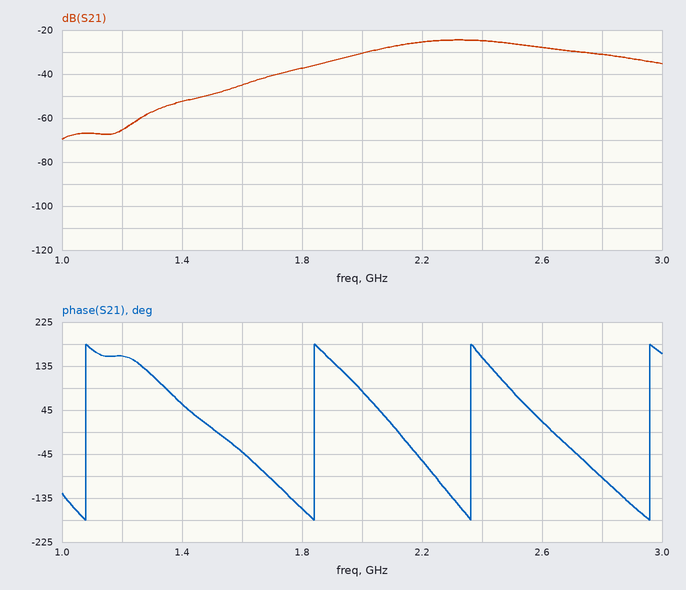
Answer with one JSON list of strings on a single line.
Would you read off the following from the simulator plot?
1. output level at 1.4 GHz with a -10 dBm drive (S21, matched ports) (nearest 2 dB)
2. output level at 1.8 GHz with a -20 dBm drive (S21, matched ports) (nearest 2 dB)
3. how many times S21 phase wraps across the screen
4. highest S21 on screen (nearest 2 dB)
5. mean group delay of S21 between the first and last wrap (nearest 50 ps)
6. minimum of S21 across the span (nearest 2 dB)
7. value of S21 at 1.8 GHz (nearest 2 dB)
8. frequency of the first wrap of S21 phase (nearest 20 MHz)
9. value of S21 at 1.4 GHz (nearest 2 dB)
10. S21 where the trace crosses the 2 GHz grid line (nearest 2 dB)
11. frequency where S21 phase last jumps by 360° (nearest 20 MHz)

["-62 dBm", "-58 dBm", "4", "-24 dB", "1.60 ns", "-70 dB", "-38 dB", "1.08 GHz", "-52 dB", "-30 dB", "2.96 GHz"]
